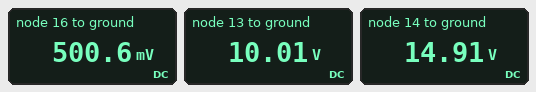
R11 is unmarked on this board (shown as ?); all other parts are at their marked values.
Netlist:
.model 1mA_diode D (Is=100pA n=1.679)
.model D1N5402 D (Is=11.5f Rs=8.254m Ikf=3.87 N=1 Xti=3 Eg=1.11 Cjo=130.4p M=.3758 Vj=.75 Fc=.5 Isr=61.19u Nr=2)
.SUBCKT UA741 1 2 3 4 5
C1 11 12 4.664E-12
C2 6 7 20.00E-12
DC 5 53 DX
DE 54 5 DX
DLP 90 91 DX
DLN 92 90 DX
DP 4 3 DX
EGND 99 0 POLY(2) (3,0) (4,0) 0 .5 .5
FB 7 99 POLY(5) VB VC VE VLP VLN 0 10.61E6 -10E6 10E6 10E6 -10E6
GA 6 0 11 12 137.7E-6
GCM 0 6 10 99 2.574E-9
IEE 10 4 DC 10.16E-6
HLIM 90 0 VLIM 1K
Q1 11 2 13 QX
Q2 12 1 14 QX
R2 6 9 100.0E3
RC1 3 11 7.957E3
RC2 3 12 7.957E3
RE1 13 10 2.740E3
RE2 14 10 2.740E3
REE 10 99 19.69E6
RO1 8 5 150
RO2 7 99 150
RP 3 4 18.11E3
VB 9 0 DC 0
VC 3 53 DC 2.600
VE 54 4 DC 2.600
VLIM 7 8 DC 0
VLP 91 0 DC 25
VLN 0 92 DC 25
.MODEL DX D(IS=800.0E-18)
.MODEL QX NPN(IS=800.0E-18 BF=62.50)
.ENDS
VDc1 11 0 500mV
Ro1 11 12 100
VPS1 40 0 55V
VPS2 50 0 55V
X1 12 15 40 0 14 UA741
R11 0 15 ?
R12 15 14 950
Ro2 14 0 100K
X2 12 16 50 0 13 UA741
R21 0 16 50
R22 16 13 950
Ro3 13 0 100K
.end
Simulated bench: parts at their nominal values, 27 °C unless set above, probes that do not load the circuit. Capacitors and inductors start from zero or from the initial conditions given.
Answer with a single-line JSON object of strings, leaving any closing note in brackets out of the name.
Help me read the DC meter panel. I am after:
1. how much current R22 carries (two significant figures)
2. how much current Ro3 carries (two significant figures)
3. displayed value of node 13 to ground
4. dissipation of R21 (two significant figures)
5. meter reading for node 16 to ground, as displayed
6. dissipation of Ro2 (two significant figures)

{"how much current R22 carries": "10 mA", "how much current Ro3 carries": "100 µA", "displayed value of node 13 to ground": "10.01 V", "dissipation of R21": "5.0 mW", "meter reading for node 16 to ground, as displayed": "500.6 mV", "dissipation of Ro2": "2.2 mW"}
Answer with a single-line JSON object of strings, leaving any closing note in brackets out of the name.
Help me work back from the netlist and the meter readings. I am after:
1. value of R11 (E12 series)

{"value of R11": "33 Ω"}
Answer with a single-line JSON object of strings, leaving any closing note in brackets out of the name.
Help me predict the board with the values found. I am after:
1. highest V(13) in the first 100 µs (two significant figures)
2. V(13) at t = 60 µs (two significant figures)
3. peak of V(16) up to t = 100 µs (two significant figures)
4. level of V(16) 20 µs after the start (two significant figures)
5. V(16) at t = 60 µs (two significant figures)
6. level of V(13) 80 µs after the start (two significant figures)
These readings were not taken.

{"highest V(13) in the first 100 µs": "10 V", "V(13) at t = 60 µs": "10 V", "peak of V(16) up to t = 100 µs": "500 mV", "level of V(16) 20 µs after the start": "450 mV", "V(16) at t = 60 µs": "500 mV", "level of V(13) 80 µs after the start": "10 V"}
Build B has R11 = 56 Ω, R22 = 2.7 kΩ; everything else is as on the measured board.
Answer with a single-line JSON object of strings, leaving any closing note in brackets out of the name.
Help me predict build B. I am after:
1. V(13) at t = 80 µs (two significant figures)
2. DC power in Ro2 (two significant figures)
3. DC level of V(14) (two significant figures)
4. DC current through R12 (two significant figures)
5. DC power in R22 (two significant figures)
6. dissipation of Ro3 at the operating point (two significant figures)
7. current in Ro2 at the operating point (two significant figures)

{"V(13) at t = 80 µs": "27 V", "DC power in Ro2": "810 µW", "DC level of V(14)": "9.0 V", "DC current through R12": "8.9 mA", "DC power in R22": "270 mW", "dissipation of Ro3 at the operating point": "7.6 mW", "current in Ro2 at the operating point": "90 µA"}
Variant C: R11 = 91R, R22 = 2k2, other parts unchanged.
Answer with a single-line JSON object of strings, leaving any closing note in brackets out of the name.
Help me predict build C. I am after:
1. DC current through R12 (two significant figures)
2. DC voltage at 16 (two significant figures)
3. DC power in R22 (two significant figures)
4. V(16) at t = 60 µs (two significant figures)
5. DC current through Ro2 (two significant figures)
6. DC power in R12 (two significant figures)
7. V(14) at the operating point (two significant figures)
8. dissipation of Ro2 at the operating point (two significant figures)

{"DC current through R12": "5.5 mA", "DC voltage at 16": "500 mV", "DC power in R22": "220 mW", "V(16) at t = 60 µs": "490 mV", "DC current through Ro2": "57 µA", "DC power in R12": "29 mW", "V(14) at the operating point": "5.7 V", "dissipation of Ro2 at the operating point": "330 µW"}
